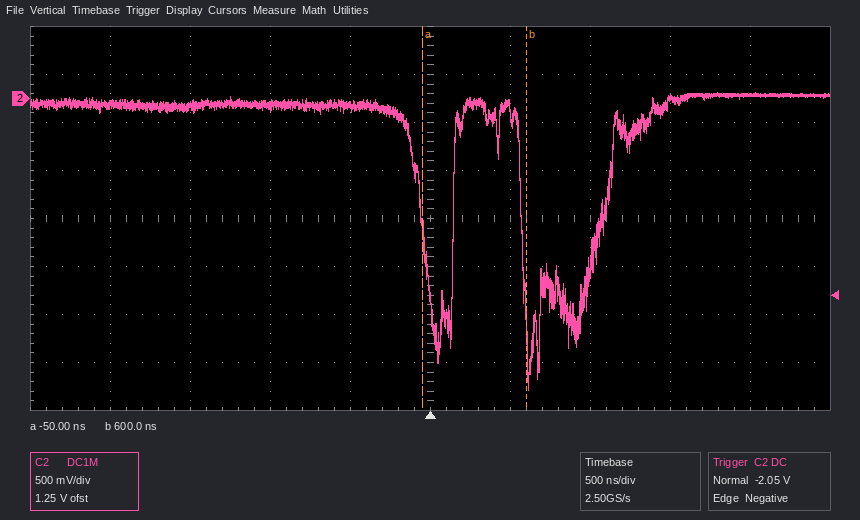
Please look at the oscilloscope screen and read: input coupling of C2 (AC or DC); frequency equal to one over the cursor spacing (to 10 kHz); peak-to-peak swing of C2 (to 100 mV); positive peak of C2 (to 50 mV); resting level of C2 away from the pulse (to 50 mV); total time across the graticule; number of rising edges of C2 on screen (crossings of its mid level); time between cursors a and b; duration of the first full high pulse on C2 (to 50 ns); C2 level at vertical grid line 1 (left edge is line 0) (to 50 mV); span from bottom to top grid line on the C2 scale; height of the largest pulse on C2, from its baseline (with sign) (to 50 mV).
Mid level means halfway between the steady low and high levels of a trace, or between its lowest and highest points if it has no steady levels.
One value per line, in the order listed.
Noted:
DC
1.54 MHz
3.10 V
50 mV
-50 mV
5 µs
2
650 ns
450 ns
-50 mV
4 V
-2.95 V
